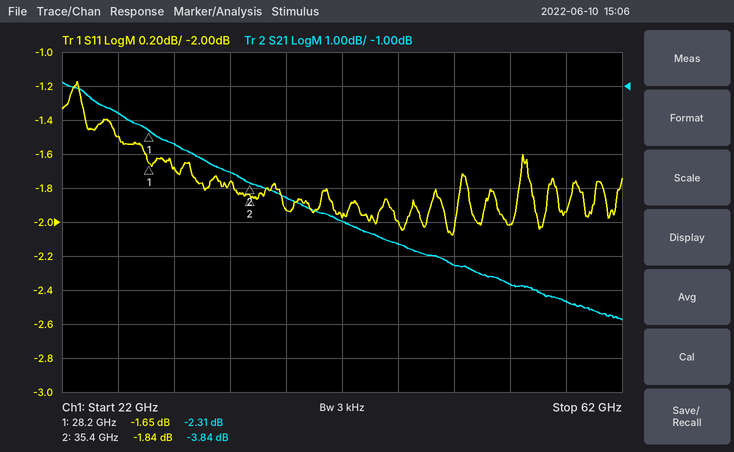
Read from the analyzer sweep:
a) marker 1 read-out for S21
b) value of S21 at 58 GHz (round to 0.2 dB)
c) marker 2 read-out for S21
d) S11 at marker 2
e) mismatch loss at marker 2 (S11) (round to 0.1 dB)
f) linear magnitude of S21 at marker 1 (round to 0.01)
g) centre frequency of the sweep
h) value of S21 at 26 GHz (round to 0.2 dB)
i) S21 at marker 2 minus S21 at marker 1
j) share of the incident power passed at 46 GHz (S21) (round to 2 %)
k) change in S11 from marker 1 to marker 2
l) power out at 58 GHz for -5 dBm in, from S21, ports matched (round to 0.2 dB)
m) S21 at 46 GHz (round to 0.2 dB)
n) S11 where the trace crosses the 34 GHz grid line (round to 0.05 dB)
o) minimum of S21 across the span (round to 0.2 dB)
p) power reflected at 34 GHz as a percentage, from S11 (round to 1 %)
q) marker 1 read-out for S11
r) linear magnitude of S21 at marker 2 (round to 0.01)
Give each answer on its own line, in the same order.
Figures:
-2.31 dB
-7.4 dB
-3.84 dB
-1.84 dB
4.6 dB
0.77
42 GHz
-1.8 dB
-1.53 dB
28 %
-0.19 dB
-12.4 dBm
-5.6 dB
-1.75 dB
-7.8 dB
67 %
-1.65 dB
0.64
